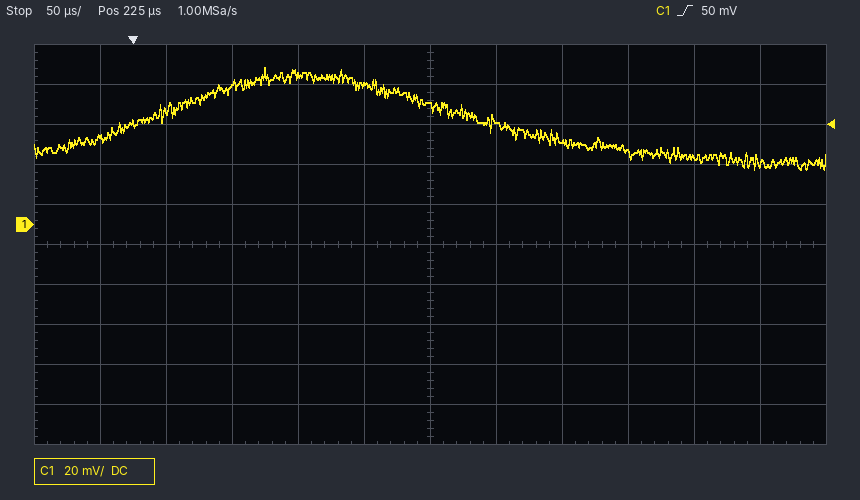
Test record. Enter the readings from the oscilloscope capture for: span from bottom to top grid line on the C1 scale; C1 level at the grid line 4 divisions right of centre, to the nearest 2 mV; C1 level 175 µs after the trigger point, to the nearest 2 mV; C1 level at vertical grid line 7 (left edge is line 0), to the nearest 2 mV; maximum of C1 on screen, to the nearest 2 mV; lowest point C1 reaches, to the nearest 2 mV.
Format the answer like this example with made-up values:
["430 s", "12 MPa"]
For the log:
["200 mV", "34 mV", "70 mV", "52 mV", "78 mV", "28 mV"]
